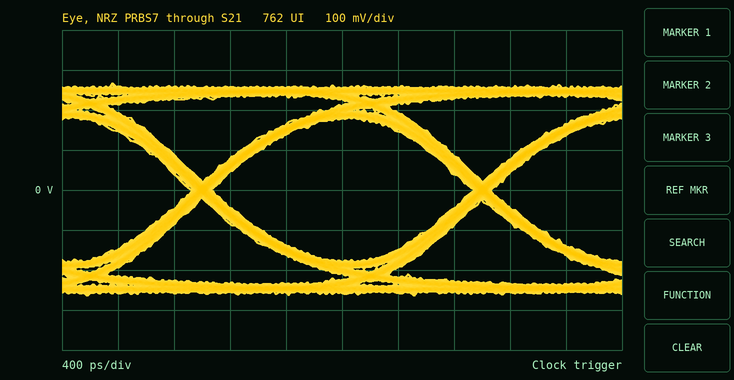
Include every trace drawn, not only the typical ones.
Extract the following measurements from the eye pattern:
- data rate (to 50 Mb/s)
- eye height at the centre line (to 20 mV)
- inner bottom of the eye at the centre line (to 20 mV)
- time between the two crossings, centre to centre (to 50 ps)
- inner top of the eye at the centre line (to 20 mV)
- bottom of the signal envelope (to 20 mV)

500 Mb/s
360 mV
-180 mV
2.00 ns
180 mV
-260 mV
